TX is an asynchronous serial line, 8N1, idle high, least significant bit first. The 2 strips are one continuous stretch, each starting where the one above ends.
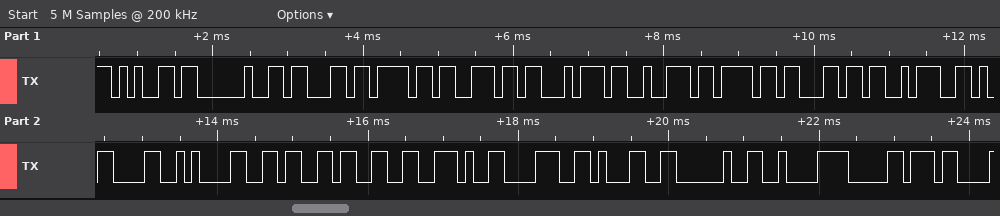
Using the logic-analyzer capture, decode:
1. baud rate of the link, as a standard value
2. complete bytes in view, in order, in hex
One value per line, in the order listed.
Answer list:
9600 baud
65 20 63 6F 6E 74 72 6F 6C 3A 0D 0A 36 33 2E 38 31 20 C2 B0
